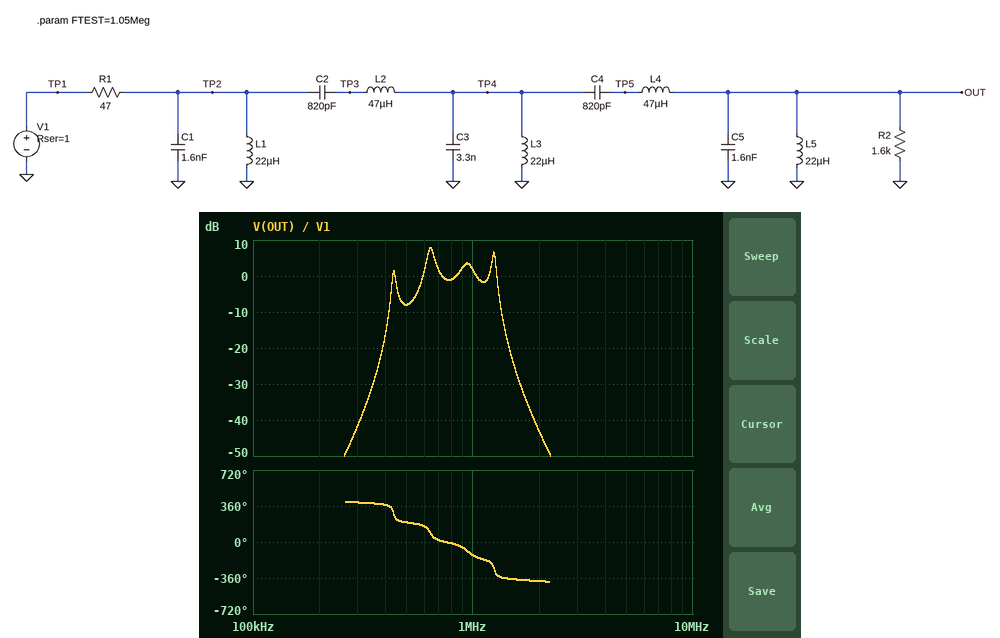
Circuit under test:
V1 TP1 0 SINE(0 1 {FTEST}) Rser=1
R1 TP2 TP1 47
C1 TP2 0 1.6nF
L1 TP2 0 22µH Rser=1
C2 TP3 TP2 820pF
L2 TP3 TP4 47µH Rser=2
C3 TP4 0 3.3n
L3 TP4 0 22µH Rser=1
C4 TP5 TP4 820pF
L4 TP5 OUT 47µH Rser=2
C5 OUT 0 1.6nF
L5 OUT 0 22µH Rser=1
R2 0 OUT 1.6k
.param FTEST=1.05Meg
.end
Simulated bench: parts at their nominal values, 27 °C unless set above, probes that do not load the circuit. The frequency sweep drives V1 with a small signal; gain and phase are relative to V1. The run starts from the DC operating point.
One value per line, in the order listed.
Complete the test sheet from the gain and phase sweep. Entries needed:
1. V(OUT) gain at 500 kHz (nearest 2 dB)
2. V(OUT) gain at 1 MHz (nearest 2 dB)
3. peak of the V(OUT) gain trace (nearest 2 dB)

-8 dB
2 dB
8 dB
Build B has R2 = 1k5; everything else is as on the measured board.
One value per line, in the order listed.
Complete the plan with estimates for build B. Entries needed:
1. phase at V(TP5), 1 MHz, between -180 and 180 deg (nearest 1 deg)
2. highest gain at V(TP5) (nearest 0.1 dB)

-82 deg
13.2 dB
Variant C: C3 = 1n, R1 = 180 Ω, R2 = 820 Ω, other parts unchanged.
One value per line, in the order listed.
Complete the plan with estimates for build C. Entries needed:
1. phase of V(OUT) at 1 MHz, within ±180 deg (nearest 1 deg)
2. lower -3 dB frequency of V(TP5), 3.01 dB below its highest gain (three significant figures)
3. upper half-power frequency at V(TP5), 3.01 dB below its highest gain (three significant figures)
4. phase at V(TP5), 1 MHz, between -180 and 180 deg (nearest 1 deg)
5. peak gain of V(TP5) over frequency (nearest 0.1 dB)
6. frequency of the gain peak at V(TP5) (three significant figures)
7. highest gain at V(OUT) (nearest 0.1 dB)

-56 deg
1.67 MHz
1.72 MHz
10 deg
12.2 dB
1.69 MHz
-0.3 dB
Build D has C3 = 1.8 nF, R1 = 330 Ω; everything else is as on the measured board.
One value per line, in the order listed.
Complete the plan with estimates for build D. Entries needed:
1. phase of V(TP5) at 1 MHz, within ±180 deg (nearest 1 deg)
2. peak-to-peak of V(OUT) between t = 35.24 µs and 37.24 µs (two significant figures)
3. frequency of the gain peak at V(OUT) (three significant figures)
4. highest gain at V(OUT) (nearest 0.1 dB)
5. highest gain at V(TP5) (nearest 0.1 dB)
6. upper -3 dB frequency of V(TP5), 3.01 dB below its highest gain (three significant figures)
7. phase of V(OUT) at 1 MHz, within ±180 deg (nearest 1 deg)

-35 deg
1.0 V
1.16 MHz
-2.0 dB
7.0 dB
1.45 MHz
-86 deg
